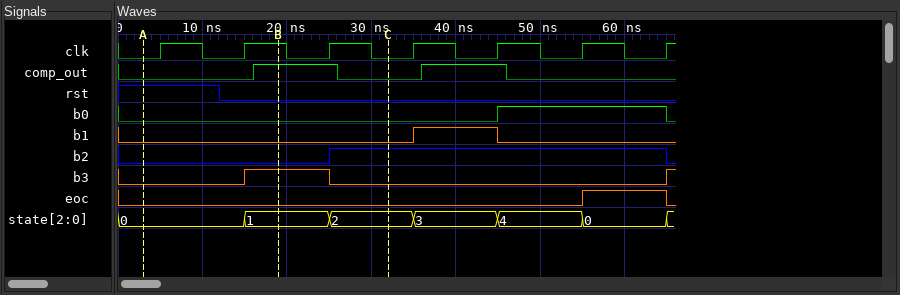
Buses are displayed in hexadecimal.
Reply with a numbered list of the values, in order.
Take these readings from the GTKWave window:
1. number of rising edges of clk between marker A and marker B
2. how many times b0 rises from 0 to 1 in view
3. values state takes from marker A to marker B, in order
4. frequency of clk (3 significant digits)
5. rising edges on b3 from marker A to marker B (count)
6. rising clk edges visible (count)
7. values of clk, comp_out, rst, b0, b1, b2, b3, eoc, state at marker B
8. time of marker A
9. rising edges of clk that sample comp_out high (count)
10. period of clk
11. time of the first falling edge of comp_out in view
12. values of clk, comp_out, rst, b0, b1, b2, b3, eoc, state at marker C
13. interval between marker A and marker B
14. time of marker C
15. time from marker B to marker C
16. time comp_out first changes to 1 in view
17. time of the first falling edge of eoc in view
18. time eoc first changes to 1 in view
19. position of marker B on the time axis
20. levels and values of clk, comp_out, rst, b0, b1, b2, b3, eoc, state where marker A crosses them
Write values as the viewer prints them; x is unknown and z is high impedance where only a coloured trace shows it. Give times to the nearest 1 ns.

1. 2
2. 1
3. 0, 1
4. 100 MHz
5. 1
6. 7
7. clk=1, comp_out=1, rst=0, b0=0, b1=0, b2=0, b3=1, eoc=0, state=1
8. 3 ns
9. 2
10. 10 ns
11. 26 ns
12. clk=0, comp_out=0, rst=0, b0=0, b1=0, b2=1, b3=0, eoc=0, state=2
13. 16 ns
14. 32 ns
15. 13 ns
16. 16 ns
17. 65 ns
18. 55 ns
19. 19 ns
20. clk=0, comp_out=0, rst=1, b0=0, b1=0, b2=0, b3=0, eoc=0, state=0
